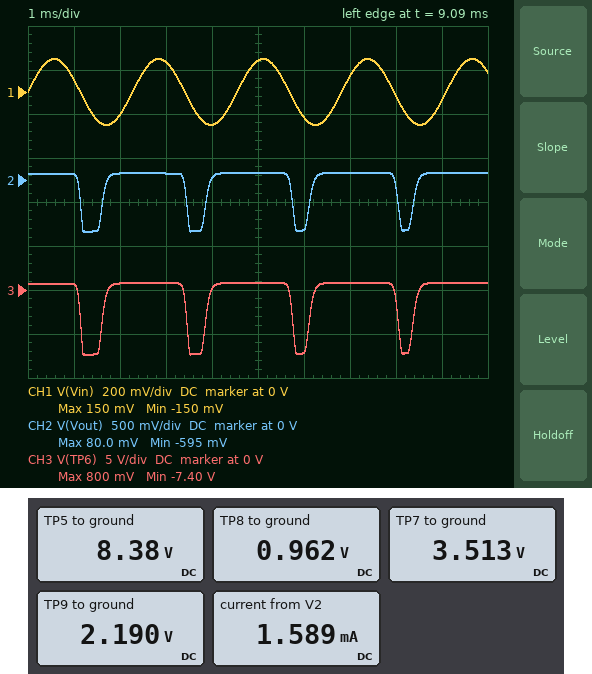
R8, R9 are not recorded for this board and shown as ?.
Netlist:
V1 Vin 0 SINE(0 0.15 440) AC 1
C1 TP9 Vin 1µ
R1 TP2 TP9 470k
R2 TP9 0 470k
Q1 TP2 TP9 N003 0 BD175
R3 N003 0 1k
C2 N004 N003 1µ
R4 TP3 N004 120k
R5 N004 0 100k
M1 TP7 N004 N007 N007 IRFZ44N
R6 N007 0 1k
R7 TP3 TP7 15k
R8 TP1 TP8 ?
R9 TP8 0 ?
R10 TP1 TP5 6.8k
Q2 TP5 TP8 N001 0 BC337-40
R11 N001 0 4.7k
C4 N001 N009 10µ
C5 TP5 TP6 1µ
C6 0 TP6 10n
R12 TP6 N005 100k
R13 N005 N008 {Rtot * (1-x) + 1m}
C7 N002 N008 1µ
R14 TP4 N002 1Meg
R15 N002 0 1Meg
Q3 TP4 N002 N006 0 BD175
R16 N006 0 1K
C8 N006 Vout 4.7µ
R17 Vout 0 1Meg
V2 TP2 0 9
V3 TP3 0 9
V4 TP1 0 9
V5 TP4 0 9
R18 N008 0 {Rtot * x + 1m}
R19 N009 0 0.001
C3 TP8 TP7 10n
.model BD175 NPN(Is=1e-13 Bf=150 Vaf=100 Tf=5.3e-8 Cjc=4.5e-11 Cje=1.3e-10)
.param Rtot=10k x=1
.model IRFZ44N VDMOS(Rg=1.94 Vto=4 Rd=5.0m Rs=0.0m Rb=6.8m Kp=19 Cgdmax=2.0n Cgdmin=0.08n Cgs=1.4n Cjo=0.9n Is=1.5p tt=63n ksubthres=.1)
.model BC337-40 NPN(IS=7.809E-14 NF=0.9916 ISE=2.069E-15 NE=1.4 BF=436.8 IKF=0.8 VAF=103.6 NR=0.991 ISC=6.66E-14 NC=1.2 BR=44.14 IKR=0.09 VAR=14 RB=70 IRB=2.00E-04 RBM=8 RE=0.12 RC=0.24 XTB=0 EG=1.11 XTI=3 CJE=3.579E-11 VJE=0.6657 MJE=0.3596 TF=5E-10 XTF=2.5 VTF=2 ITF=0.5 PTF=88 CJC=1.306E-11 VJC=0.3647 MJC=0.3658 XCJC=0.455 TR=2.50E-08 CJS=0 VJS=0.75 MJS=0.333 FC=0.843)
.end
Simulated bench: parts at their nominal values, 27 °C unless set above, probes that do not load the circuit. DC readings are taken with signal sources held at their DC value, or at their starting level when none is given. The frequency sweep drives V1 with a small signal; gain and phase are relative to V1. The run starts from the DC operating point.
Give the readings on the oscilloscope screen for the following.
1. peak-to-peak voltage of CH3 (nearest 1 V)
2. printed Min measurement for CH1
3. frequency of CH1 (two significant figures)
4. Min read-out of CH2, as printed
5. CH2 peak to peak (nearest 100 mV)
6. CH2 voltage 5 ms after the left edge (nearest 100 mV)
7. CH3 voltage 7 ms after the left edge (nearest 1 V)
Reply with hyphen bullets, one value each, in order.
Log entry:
- 8 V
- -150 mV
- 440 Hz
- -595 mV
- 700 mV
- 100 mV
- 1 V
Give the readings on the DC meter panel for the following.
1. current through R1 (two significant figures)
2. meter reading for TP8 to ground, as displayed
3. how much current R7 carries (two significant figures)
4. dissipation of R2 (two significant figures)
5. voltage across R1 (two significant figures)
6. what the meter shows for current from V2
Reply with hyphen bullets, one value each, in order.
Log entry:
- 14 µA
- 0.962 V
- 370 µA
- 10 µW
- 6.8 V
- 1.589 mA
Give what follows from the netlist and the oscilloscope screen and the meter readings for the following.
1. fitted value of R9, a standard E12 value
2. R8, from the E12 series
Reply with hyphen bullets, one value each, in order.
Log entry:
- 12 kΩ
- 100 kΩ
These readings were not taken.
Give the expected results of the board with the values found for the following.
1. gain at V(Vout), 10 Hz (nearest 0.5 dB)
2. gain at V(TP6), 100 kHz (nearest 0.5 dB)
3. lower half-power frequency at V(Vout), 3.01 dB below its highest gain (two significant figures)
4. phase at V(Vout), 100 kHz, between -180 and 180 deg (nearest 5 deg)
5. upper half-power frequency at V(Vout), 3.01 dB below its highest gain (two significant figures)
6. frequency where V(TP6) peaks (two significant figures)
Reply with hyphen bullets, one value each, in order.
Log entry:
- -32.0 dB
- -3.0 dB
- 430 Hz
- 115 deg
- 3.4 kHz
- 1.2 kHz
